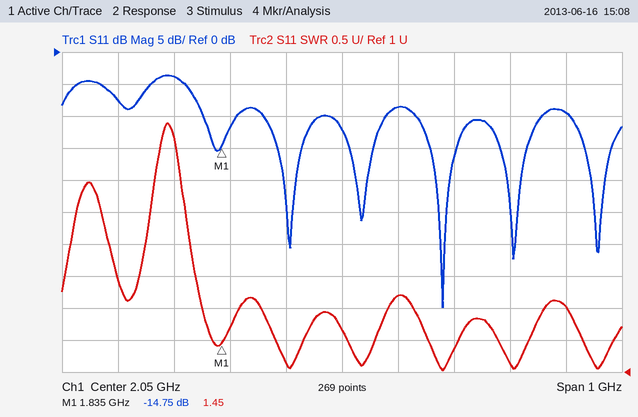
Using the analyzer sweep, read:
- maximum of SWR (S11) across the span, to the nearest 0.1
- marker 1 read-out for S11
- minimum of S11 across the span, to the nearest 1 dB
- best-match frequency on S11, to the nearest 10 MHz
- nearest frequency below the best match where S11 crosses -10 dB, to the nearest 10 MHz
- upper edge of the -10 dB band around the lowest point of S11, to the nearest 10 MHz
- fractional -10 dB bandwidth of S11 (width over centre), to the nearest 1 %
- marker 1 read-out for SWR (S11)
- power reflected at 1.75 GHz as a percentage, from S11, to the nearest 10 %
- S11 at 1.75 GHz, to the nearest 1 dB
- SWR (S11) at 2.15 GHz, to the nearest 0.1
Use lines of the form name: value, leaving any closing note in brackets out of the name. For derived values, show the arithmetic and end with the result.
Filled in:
maximum of SWR (S11) across the span, to the nearest 0.1: 4.9
marker 1 read-out for S11: -14.75 dB
minimum of S11 across the span, to the nearest 1 dB: -40 dB
best-match frequency on S11, to the nearest 10 MHz: 2.23 GHz
nearest frequency below the best match where S11 crosses -10 dB, to the nearest 10 MHz: 2.18 GHz
upper edge of the -10 dB band around the lowest point of S11, to the nearest 10 MHz: 2.41 GHz
fractional -10 dB bandwidth of S11 (width over centre), to the nearest 1 %: 230 MHz / 2.295 GHz ≈ 10 %
marker 1 read-out for SWR: 1.45
power reflected at 1.75 GHz as a percentage, from S11, to the nearest 10 %: 10^(-4/10) ≈ 40 %
S11 at 1.75 GHz, to the nearest 1 dB: -4 dB
SWR (S11) at 2.15 GHz, to the nearest 0.1: 2.2
